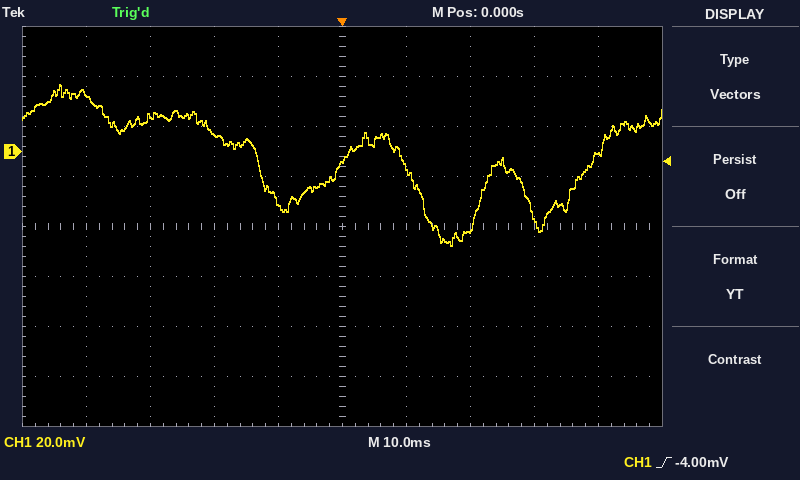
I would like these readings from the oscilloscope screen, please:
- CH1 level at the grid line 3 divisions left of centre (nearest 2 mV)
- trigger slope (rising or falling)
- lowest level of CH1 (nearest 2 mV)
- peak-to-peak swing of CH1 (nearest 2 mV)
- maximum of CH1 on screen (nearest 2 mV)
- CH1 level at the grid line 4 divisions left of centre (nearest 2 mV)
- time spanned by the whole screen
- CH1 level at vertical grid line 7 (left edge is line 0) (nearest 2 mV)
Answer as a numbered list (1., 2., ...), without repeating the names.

1. 14 mV
2. rising
3. -38 mV
4. 64 mV
5. 26 mV
6. 24 mV
7. 100 ms
8. -30 mV
